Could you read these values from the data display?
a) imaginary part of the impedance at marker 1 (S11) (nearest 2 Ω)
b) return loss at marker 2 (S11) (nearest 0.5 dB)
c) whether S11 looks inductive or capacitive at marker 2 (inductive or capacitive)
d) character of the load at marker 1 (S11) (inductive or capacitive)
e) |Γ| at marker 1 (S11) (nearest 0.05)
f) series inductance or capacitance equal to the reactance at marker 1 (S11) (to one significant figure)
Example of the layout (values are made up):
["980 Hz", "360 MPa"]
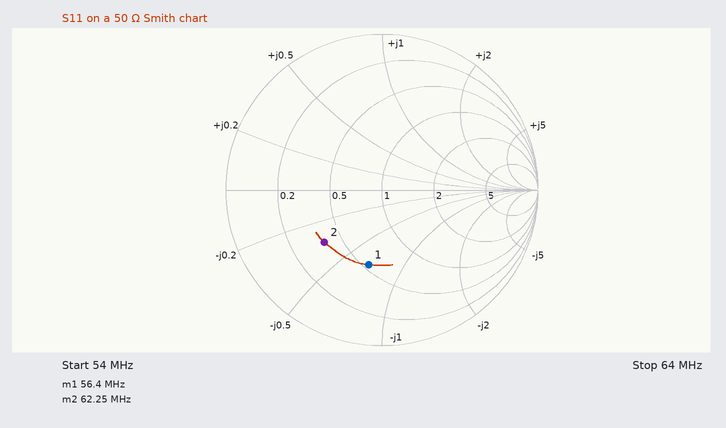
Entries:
["-34 Ω", "6.0 dB", "capacitive", "capacitive", "0.50", "80 pF"]
